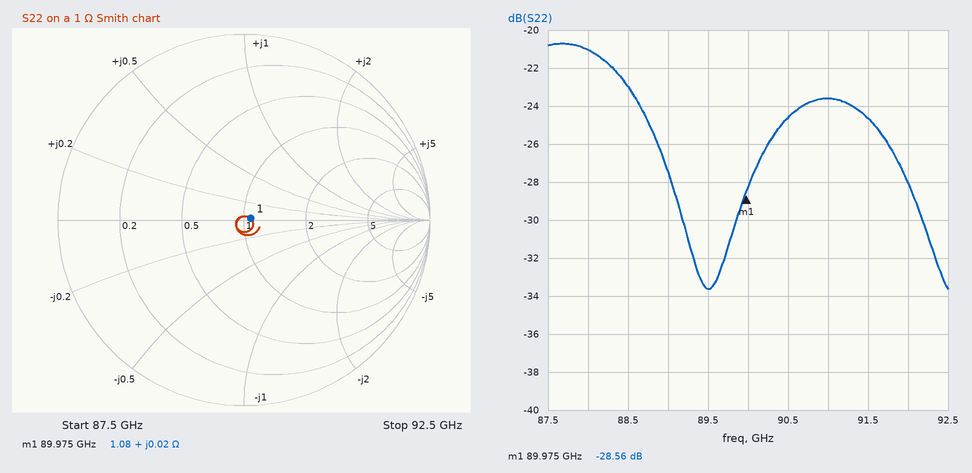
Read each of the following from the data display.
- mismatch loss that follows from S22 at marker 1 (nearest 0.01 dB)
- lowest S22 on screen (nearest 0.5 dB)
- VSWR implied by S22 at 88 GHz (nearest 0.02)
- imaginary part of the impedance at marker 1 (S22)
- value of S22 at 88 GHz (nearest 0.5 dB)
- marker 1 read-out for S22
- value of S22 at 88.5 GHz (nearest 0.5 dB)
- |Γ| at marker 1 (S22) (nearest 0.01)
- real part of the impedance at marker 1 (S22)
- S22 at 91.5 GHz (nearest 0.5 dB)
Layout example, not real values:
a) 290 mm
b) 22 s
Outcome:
a) 0.01 dB
b) -33.5 dB
c) 1.20
d) +0.02 Ω
e) -21.0 dB
f) -28.56 dB
g) -23.0 dB
h) 0.04
i) 1.08 Ω
j) -24.5 dB
